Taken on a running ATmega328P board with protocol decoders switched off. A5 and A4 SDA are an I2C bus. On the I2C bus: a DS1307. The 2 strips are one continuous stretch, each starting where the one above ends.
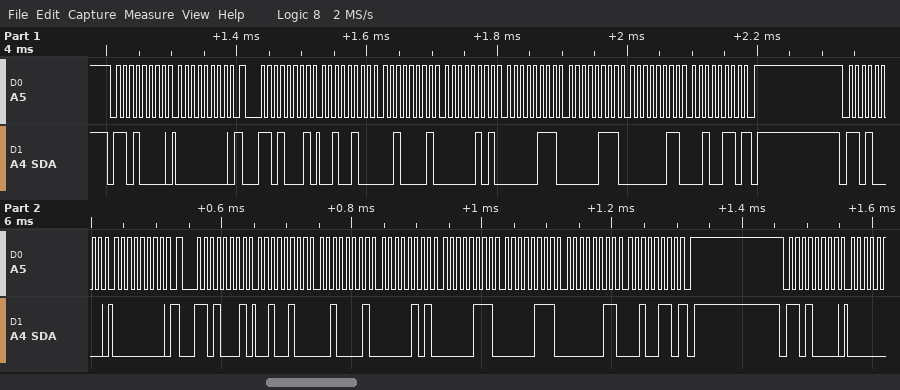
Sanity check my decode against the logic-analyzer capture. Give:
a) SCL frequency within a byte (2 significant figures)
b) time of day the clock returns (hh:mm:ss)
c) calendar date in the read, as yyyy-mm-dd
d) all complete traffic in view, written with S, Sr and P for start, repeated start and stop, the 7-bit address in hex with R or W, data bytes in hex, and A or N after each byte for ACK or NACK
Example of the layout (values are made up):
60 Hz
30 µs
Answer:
100 kHz
05:21:24
2026-03-07
S 68W A 00 A Sr 68R A 24 A 21 A 05 A 07 A 07 A 03 A 26 N P S 68W A 00 A Sr 68R A 24 A 21 A 05 A 07 A 07 A 03 A 26 N P S 68W A
